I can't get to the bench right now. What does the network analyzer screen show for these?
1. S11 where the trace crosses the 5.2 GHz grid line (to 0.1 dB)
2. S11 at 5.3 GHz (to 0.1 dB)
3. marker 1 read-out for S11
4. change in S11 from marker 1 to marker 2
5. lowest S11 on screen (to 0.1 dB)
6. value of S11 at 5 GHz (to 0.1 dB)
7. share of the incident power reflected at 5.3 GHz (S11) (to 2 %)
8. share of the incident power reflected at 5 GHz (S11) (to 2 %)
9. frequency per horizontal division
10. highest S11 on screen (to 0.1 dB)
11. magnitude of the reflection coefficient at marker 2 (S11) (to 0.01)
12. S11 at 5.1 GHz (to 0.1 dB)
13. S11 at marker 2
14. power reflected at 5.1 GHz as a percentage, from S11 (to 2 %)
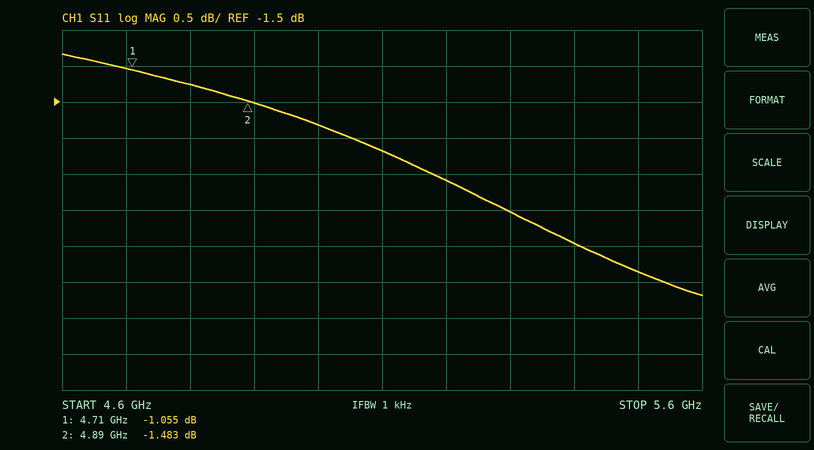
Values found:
-2.6 dB
-3.0 dB
-1.055 dB
-0.428 dB
-4.2 dB
-1.8 dB
50 %
66 %
100 MHz
-0.8 dB
0.84
-2.2 dB
-1.483 dB
60 %
